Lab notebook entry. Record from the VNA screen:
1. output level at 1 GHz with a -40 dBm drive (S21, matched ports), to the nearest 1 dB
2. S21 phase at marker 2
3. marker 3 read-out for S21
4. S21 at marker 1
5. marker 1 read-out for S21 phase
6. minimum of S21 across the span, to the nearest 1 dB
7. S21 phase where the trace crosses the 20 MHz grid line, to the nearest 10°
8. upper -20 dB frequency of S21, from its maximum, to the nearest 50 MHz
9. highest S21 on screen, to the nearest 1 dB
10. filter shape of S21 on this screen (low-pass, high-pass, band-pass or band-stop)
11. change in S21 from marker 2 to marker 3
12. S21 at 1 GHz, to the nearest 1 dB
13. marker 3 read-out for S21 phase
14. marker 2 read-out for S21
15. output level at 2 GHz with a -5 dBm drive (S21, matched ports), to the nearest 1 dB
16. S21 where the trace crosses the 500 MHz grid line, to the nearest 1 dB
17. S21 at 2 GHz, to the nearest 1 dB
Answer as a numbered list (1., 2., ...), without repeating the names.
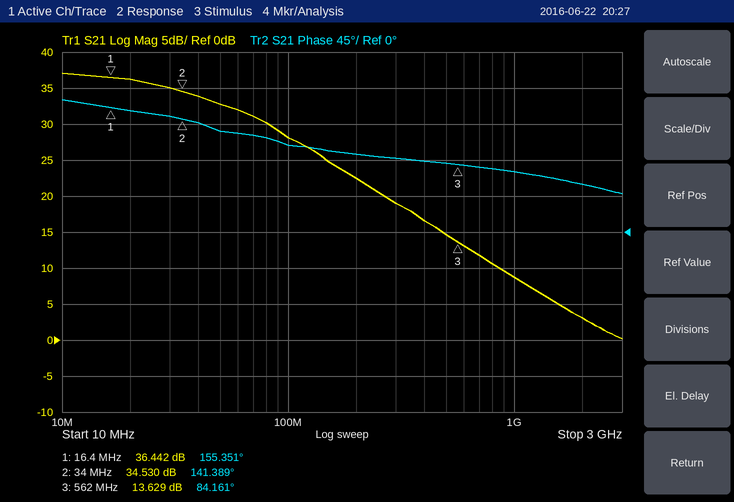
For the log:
1. -31 dBm
2. 141.389°
3. 13.629 dB
4. 36.442 dB
5. 155.351°
6. 0 dB
7. 150°
8. 400 MHz
9. 37 dB
10. low-pass
11. -20.901 dB
12. 9 dB
13. 84.161°
14. 34.530 dB
15. -2 dBm
16. 15 dB
17. 3 dB
